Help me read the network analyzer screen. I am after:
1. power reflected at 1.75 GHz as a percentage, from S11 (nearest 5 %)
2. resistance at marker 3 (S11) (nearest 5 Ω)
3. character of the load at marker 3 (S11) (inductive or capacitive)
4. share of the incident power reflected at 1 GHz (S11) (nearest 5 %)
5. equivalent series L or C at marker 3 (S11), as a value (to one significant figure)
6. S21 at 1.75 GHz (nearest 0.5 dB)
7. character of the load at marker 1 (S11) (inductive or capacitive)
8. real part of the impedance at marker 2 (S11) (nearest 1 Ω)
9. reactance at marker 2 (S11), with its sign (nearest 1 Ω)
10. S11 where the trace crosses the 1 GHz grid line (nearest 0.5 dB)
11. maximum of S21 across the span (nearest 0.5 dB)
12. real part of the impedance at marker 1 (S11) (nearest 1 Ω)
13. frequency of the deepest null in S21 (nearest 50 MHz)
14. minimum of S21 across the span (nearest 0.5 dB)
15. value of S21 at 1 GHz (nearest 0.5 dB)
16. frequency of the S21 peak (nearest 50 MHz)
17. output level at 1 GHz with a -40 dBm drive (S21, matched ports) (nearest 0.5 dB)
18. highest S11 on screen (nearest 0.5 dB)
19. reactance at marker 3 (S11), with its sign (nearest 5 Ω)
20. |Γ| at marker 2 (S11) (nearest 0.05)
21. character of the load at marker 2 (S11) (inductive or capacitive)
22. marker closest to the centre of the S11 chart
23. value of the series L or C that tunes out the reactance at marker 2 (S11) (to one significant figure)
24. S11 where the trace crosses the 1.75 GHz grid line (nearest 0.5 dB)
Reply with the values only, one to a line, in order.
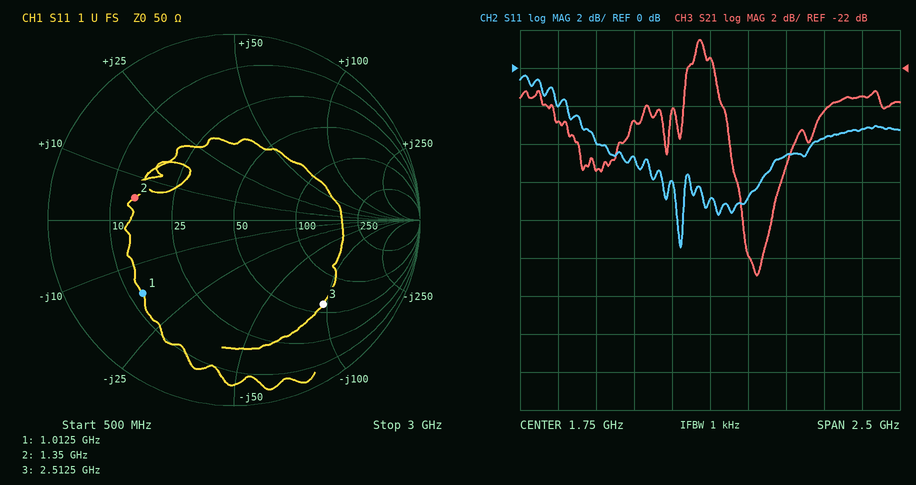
20 %
60 Ω
capacitive
40 %
700 fF
-21.5 dB
capacitive
15 Ω
+5 Ω
-4.0 dB
-20.5 dB
13 Ω
2.05 GHz
-33.0 dB
-27.5 dB
1.70 GHz
-67.5 dBm
-0.5 dB
-95 Ω
0.55
inductive
marker 2
20 pF
-7.0 dB
